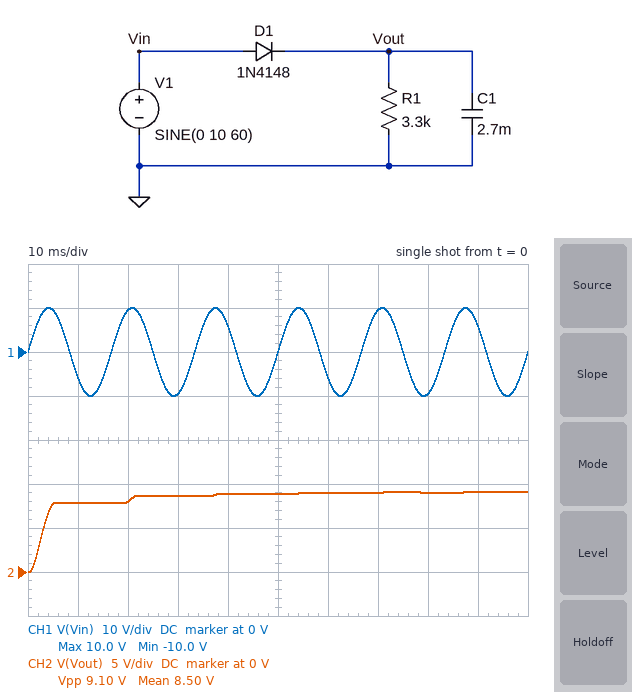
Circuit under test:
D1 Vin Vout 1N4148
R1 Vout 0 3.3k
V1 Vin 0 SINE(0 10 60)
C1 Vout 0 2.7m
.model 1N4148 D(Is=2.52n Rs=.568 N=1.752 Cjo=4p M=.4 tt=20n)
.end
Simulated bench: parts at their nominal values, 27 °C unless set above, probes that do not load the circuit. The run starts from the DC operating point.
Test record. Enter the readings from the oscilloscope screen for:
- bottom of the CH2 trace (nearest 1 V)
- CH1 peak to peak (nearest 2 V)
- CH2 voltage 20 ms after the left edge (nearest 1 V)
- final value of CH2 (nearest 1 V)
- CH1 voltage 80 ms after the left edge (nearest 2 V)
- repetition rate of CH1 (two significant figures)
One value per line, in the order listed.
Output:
0 V
20 V
8 V
9 V
-10 V
60 Hz
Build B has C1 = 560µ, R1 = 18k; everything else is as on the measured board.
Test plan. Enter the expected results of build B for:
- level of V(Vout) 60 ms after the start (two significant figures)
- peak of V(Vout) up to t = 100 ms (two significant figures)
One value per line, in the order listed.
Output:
9.2 V
9.3 V
